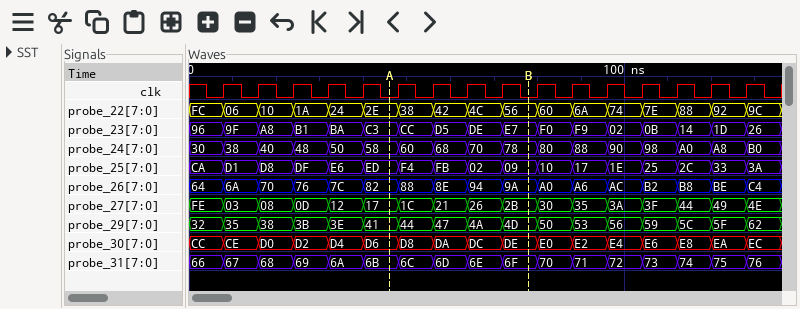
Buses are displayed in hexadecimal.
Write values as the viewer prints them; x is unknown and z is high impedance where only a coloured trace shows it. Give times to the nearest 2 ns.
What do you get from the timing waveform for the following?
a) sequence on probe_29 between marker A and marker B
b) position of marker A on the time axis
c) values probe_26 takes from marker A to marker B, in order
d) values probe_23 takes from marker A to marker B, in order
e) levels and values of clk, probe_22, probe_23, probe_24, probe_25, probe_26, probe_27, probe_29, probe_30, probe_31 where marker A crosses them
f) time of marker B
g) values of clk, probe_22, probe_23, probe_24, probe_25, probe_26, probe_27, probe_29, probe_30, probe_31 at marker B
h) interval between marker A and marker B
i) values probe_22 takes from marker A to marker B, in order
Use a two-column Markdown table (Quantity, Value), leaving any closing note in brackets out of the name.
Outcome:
| Quantity | Value |
|---|---|
| sequence on probe_29 between marker A and marker B | 41, 44, 47, 4A, 4D |
| position of marker A on the time axis | 46 ns |
| values probe_26 takes from marker A to marker B, in order | 82, 88, 8E, 94, 9A |
| values probe_23 takes from marker A to marker B, in order | C3, CC, D5, DE, E7 |
| levels and values of clk, probe_22, probe_23, probe_24, probe_25, probe_26, probe_27, probe_29, probe_30, probe_31 where marker A crosses them | clk=0, probe_22=2E, probe_23=C3, probe_24=58, probe_25=ED, probe_26=82, probe_27=17, probe_29=41, probe_30=D6, probe_31=6B |
| time of marker B | 78 ns |
| values of clk, probe_22, probe_23, probe_24, probe_25, probe_26, probe_27, probe_29, probe_30, probe_31 at marker B | clk=0, probe_22=56, probe_23=E7, probe_24=78, probe_25=09, probe_26=9A, probe_27=2B, probe_29=4D, probe_30=DE, probe_31=6F |
| interval between marker A and marker B | 32 ns |
| values probe_22 takes from marker A to marker B, in order | 2E, 38, 42, 4C, 56 |
